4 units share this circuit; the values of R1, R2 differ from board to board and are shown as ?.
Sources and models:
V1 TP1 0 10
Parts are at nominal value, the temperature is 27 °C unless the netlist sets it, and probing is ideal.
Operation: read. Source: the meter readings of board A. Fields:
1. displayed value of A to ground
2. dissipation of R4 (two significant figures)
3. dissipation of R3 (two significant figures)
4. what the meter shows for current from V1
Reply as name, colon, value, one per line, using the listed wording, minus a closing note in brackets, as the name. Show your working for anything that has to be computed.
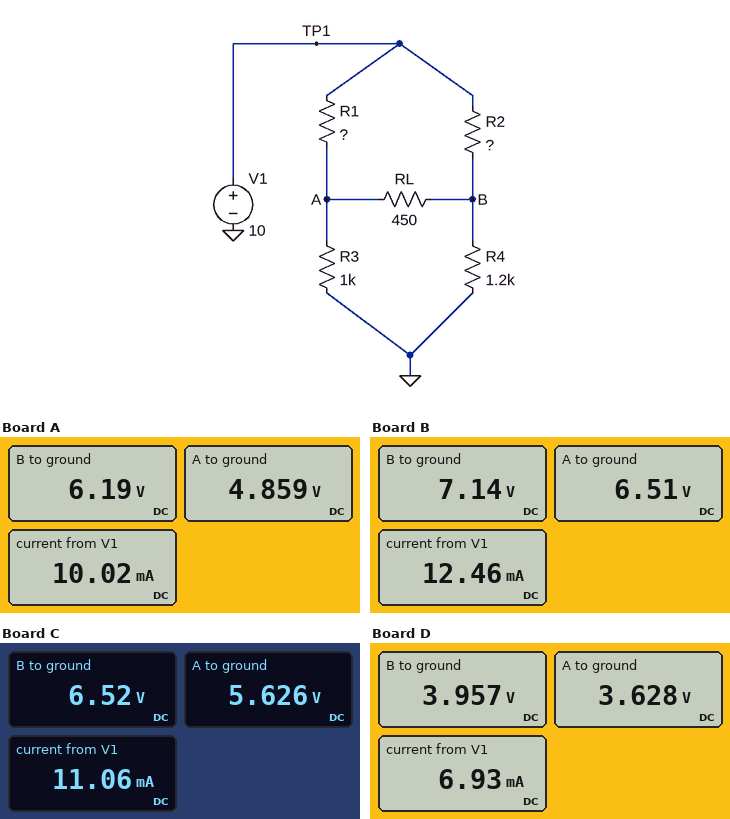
displayed value of A to ground: 4.859 V
dissipation of R4: (6.19 V)^2 / 1.2 kΩ = 32 mW
dissipation of R3: (4.859 V)^2 / 1 kΩ = 24 mW
what the meter shows for current from V1: 10.02 mA
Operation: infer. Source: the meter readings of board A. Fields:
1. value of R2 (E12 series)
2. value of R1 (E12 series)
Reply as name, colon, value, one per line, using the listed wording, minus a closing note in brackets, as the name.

value of R2: 470 Ω
value of R1: 2.7 kΩ
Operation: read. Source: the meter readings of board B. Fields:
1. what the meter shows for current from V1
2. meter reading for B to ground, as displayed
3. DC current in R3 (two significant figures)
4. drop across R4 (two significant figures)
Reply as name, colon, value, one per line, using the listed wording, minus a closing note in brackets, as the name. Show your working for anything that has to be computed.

what the meter shows for current from V1: 12.46 mA
meter reading for B to ground, as displayed: 7.14 V
DC current in R3: (6.51 V) / 1 kΩ = 6.5 mA
drop across R4: 7.14 V = 7.1 V
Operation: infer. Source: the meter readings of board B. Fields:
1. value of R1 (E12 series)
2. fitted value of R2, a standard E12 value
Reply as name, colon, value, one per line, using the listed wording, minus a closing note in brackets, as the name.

value of R1: 680 Ω
fitted value of R2, a standard E12 value: 390 Ω
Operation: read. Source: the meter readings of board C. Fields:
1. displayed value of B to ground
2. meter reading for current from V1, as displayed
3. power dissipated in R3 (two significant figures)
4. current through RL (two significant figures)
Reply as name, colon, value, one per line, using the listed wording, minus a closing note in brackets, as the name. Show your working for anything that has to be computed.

displayed value of B to ground: 6.52 V
meter reading for current from V1, as displayed: 11.06 mA
power dissipated in R3: (5.626 V)^2 / 1 kΩ = 32 mW
current through RL: (6.52 V - 5.626 V) / 450 Ω = 2.0 mA
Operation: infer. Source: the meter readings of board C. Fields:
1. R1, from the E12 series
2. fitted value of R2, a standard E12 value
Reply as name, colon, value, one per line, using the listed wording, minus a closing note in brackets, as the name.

R1, from the E12 series: 1.2 kΩ
fitted value of R2, a standard E12 value: 470 Ω
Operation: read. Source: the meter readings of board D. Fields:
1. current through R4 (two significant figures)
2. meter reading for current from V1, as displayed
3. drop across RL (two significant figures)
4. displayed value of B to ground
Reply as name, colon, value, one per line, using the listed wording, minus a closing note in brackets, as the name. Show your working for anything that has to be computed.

current through R4: (3.957 V) / 1.2 kΩ = 3.3 mA
meter reading for current from V1, as displayed: 6.93 mA
drop across RL: 3.957 V - 3.628 V = 330 mV
displayed value of B to ground: 3.957 V
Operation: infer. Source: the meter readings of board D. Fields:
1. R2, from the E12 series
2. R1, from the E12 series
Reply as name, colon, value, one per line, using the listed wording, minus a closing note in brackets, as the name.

R2, from the E12 series: 1.5 kΩ
R1, from the E12 series: 2.2 kΩ
